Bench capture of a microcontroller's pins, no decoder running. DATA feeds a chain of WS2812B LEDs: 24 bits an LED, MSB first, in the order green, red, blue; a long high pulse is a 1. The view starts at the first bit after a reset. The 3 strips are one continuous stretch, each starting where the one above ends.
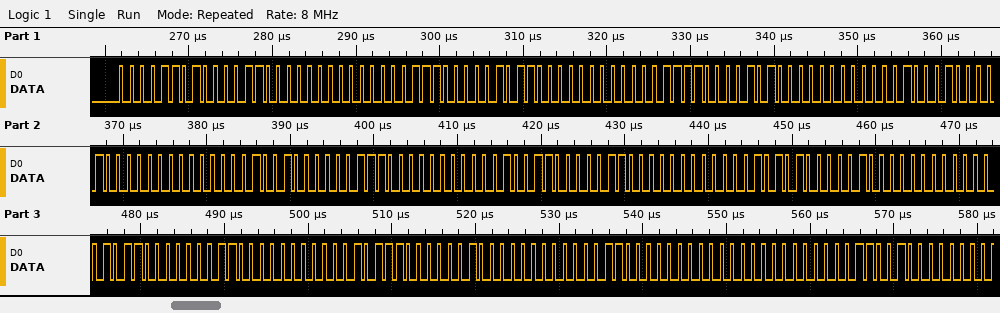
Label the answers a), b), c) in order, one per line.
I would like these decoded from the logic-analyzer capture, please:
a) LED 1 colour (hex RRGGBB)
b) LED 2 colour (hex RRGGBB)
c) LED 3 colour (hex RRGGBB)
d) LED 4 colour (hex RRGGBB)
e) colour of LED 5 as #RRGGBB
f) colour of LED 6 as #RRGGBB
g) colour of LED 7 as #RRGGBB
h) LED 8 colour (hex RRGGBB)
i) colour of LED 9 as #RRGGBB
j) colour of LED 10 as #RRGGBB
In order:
a) #0C0D00
b) #0B0E00
c) #0A0F00
d) #081100
e) #071200
f) #061300
g) #041500
h) #031600
i) #021700
j) #001800
